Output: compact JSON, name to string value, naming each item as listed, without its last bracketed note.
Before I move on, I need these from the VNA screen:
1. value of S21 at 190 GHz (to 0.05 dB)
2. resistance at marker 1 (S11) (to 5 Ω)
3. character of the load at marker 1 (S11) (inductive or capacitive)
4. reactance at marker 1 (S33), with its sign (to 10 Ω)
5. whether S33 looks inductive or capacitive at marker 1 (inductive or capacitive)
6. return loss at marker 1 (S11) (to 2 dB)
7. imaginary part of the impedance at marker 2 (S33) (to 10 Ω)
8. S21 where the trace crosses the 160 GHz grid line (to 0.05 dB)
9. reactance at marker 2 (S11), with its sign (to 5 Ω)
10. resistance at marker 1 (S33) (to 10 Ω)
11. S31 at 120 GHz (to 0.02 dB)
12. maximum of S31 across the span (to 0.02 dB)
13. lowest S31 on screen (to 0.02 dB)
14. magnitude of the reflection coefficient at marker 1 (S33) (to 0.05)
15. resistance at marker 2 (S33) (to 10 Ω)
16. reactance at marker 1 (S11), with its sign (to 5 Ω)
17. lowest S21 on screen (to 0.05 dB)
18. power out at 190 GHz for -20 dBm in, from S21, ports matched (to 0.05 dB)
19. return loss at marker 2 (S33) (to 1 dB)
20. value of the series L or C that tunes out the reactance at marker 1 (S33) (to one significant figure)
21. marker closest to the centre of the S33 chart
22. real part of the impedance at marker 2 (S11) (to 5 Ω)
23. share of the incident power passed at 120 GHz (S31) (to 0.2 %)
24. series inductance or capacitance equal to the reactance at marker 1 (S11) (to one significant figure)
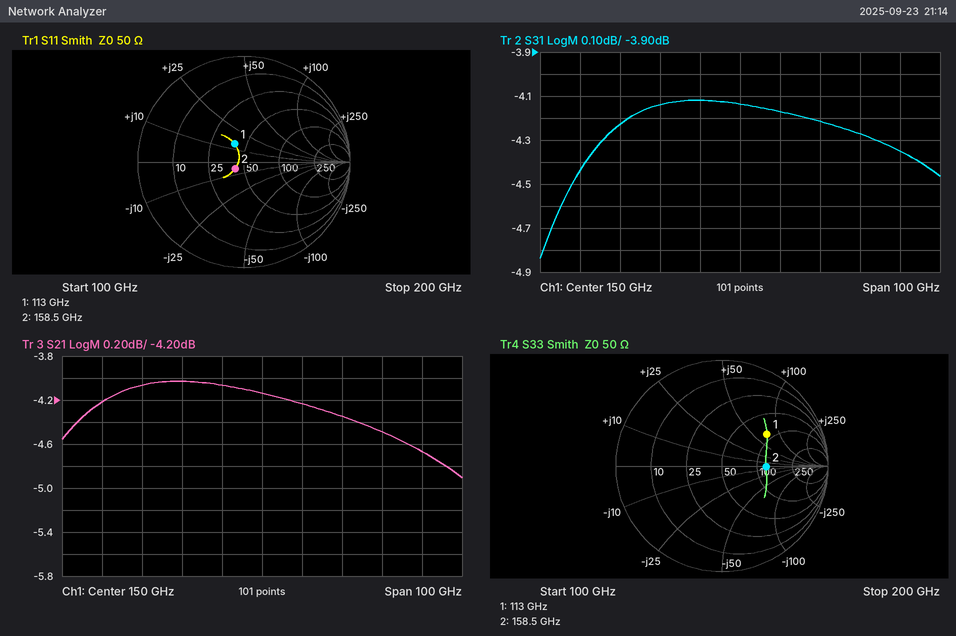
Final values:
{"value of S21 at 190 GHz": "-4.65 dB", "resistance at marker 1 (S11)": "40 Ω", "character of the load at marker 1 (S11)": "inductive", "reactance at marker 1 (S33), with its sign": "+70 Ω", "whether S33 looks inductive or capacitive at marker 1": "inductive", "return loss at marker 1 (S11)": "14 dB", "imaginary part of the impedance at marker 2 (S33)": "0 Ω", "S21 where the trace crosses the 160 GHz grid line": "-4.25 dB", "reactance at marker 2 (S11), with its sign": "-5 Ω", "resistance at marker 1 (S33)": "90 Ω", "S31 at 120 GHz": "-4.22 dB", "maximum of S31 across the span": "-4.12 dB", "lowest S31 on screen": "-4.84 dB", "magnitude of the reflection coefficient at marker 1 (S33)": "0.50", "resistance at marker 2 (S33)": "120 Ω", "reactance at marker 1 (S11), with its sign": "+15 Ω", "lowest S21 on screen": "-4.90 dB", "power out at 190 GHz for -20 dBm in, from S21, ports matched": "-24.65 dBm", "return loss at marker 2 (S33)": "8 dB", "value of the series L or C that tunes out the reactance at marker 1 (S33)": "20 fF", "marker closest to the centre of the S33 chart": "marker 2", "real part of the impedance at marker 2 (S11)": "40 Ω", "share of the incident power passed at 120 GHz (S31)": "37.8 %", "series inductance or capacitance equal to the reactance at marker 1 (S11)": "20 pH"}
